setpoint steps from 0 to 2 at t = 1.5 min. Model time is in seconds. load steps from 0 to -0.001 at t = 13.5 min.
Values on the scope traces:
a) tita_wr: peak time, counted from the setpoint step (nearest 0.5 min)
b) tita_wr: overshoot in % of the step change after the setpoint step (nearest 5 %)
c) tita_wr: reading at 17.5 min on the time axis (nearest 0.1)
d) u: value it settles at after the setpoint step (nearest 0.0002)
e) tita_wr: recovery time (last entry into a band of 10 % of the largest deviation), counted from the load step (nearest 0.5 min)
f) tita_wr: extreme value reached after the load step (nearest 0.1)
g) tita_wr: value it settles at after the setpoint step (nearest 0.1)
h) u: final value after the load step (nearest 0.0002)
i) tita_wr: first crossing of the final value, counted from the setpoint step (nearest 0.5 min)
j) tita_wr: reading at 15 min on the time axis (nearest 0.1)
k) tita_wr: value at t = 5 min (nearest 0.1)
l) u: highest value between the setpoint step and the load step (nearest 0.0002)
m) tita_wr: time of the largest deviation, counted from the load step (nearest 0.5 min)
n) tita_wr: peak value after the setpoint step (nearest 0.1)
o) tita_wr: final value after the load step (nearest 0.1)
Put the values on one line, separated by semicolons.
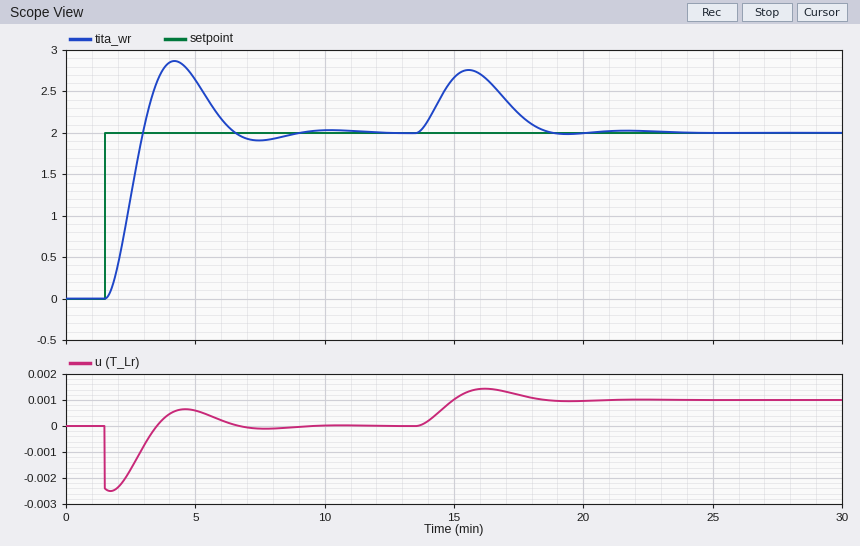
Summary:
2.5 min; 45 %; 2.2; 0.0000; 4.5 min; 2.8; 2.0; 0.0010; 1.5 min; 2.7; 2.6; 0.0006; 2.0 min; 2.9; 2.0
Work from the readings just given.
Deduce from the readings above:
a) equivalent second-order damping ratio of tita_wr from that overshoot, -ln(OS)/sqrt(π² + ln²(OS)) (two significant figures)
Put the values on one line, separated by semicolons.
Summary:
0.25
